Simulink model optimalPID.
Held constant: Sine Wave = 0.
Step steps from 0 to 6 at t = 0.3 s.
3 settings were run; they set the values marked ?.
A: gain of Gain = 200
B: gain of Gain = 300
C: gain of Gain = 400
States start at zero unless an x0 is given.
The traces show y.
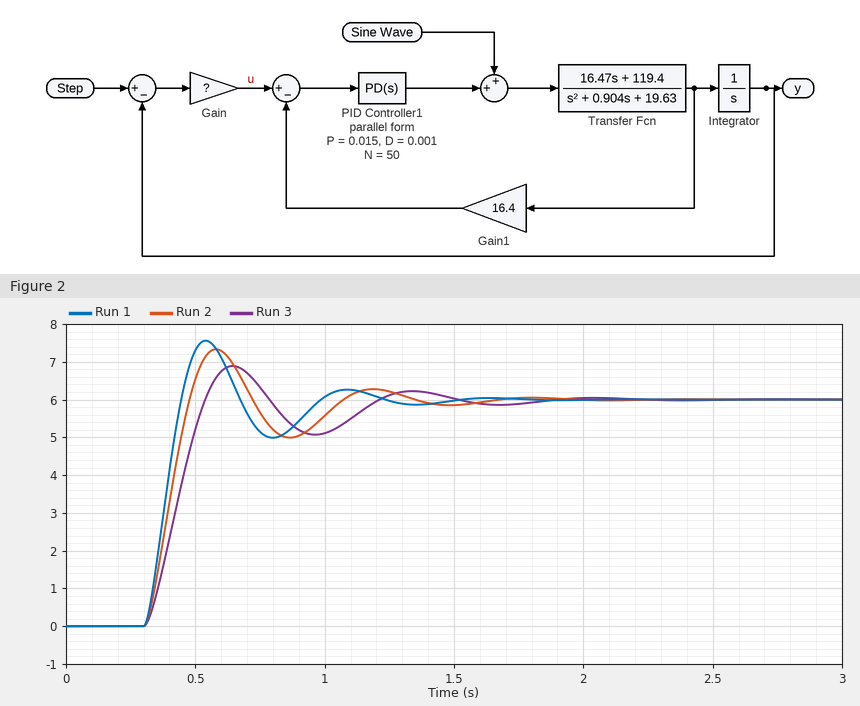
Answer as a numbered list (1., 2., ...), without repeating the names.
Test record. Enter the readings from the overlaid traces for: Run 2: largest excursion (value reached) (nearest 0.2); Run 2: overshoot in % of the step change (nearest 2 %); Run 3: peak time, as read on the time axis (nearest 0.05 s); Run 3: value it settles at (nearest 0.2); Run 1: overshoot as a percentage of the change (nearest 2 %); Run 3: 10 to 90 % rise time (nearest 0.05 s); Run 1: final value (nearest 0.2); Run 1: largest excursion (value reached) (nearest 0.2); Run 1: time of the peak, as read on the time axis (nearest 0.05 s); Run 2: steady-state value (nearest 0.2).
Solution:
1. 7.4
2. 22 %
3. 0.65 s
4. 6.0
5. 26 %
6. 0.15 s
7. 6.0
8. 7.6
9. 0.55 s
10. 6.0
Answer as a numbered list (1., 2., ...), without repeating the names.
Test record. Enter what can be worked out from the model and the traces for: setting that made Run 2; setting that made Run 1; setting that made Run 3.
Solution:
1. B
2. C
3. A
